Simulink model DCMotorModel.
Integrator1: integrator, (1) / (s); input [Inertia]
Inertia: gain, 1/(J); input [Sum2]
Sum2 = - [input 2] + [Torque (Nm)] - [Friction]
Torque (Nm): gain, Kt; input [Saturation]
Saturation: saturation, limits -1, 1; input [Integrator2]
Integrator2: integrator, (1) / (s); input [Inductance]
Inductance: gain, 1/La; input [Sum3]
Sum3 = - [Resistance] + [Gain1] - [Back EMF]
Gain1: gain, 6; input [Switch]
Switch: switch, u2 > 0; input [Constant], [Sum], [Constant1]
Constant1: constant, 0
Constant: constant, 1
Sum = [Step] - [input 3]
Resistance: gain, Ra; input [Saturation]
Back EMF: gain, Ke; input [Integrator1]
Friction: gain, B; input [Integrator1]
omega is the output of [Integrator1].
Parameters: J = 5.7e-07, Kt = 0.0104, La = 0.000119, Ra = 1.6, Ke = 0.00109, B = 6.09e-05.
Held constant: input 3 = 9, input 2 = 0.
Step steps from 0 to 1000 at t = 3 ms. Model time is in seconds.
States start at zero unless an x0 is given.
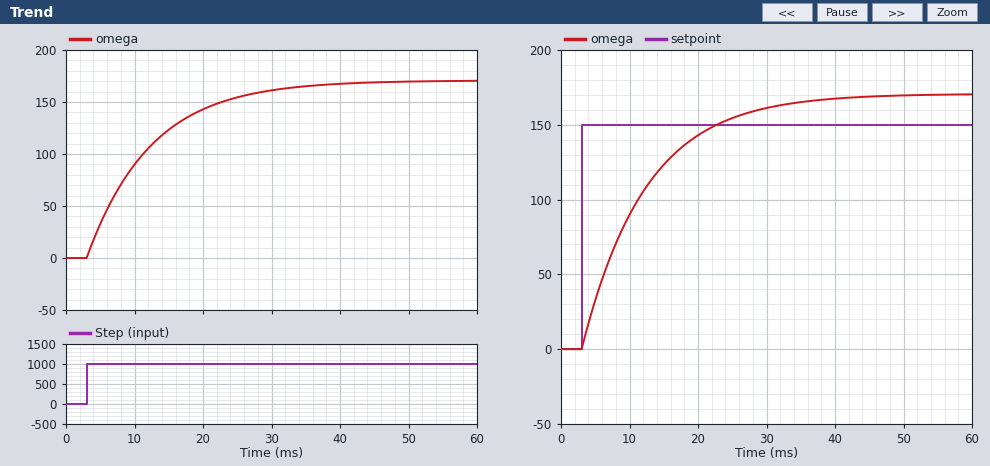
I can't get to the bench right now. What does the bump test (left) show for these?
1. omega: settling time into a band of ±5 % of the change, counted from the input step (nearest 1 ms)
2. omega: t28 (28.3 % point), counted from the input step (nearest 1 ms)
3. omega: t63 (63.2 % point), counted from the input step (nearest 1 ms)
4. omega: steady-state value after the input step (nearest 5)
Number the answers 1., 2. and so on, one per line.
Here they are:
1. 28 ms
2. 3 ms
3. 9 ms
4. 170
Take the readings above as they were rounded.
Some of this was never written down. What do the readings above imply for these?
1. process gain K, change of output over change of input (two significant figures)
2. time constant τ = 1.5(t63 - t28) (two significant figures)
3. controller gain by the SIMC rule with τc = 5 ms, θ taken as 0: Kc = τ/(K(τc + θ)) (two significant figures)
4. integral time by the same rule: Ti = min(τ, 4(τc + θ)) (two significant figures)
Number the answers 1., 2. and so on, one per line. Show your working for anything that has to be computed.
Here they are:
1. (170 - 0) / 1000 = 0.17
2. 1.5 × (9 - 3) = 9.0 ms
3. 9 / (0.17 × (5 + 0)) = 11
4. min(9, 4 × (5 + 0)) = 9.0 ms
